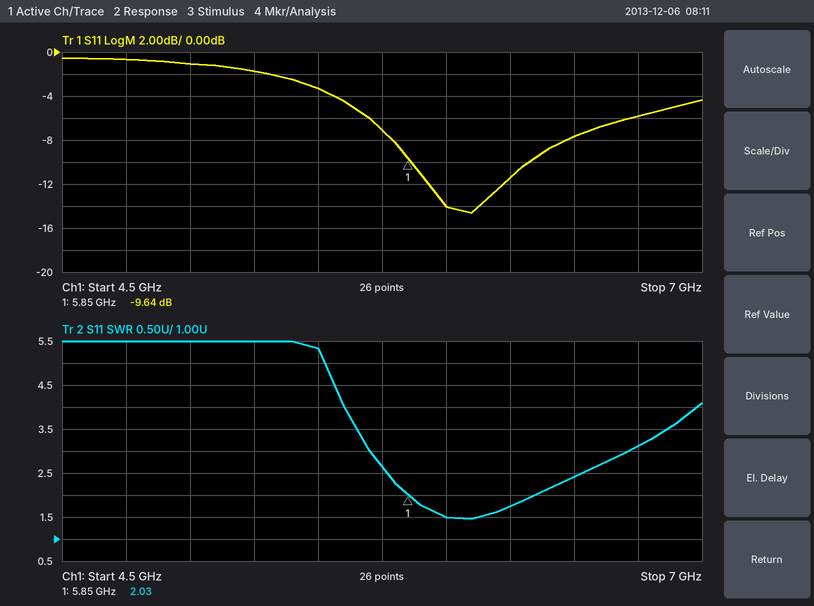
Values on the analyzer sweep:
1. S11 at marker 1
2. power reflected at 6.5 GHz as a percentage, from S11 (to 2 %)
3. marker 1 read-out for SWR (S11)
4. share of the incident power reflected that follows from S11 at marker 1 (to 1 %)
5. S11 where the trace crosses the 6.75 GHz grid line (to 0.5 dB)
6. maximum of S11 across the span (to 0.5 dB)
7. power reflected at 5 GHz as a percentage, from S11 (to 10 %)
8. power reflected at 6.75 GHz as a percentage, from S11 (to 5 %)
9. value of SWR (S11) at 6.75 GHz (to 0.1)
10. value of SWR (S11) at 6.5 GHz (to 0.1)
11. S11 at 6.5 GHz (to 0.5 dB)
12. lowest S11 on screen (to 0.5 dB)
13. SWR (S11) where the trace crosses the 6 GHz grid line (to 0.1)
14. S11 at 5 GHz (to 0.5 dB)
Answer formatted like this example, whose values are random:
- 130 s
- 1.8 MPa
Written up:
- -9.64 dB
- 18 %
- 2.03
- 11 %
- -6.0 dB
- -0.5 dB
- 80 %
- 25 %
- 3.1
- 2.4
- -7.5 dB
- -14.5 dB
- 1.5
- -1.0 dB
